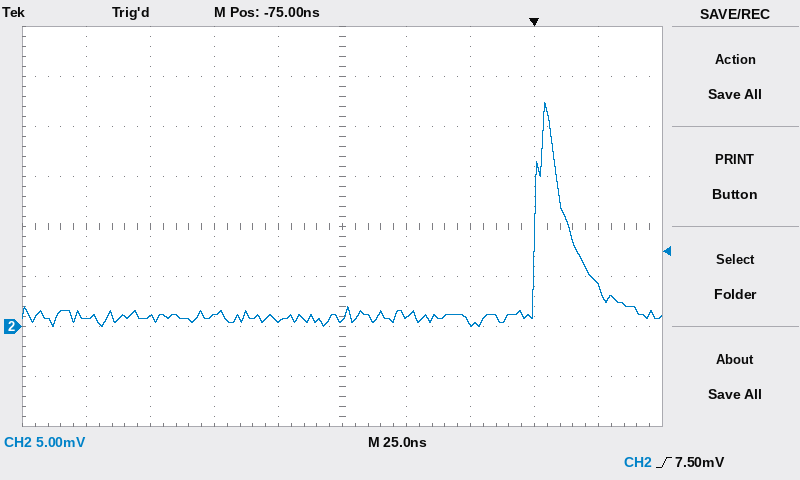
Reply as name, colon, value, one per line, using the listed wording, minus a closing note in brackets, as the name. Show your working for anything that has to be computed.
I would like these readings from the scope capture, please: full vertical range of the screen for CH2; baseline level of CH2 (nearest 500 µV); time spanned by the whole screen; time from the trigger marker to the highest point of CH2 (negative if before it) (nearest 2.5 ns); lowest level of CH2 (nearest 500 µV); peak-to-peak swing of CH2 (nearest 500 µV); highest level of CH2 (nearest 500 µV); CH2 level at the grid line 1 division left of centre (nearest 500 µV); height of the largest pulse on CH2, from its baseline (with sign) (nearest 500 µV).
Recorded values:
full vertical range of the screen for CH2: 40 mV
baseline level of CH2: 1.0 mV
time spanned by the whole screen: 250 ns
time from the trigger marker to the highest point of CH2 (negative if before it): +5.0 ns
lowest level of CH2: 0.0 mV
peak-to-peak swing of CH2: 22.5 mV − (0.0 mV) = 22.5 mV
highest level of CH2: 22.5 mV
CH2 level at the grid line 1 division left of centre: 500 µV
height of the largest pulse on CH2, from its baseline (with sign): 22.5 mV − (1.0 mV) = +21.5 mV
